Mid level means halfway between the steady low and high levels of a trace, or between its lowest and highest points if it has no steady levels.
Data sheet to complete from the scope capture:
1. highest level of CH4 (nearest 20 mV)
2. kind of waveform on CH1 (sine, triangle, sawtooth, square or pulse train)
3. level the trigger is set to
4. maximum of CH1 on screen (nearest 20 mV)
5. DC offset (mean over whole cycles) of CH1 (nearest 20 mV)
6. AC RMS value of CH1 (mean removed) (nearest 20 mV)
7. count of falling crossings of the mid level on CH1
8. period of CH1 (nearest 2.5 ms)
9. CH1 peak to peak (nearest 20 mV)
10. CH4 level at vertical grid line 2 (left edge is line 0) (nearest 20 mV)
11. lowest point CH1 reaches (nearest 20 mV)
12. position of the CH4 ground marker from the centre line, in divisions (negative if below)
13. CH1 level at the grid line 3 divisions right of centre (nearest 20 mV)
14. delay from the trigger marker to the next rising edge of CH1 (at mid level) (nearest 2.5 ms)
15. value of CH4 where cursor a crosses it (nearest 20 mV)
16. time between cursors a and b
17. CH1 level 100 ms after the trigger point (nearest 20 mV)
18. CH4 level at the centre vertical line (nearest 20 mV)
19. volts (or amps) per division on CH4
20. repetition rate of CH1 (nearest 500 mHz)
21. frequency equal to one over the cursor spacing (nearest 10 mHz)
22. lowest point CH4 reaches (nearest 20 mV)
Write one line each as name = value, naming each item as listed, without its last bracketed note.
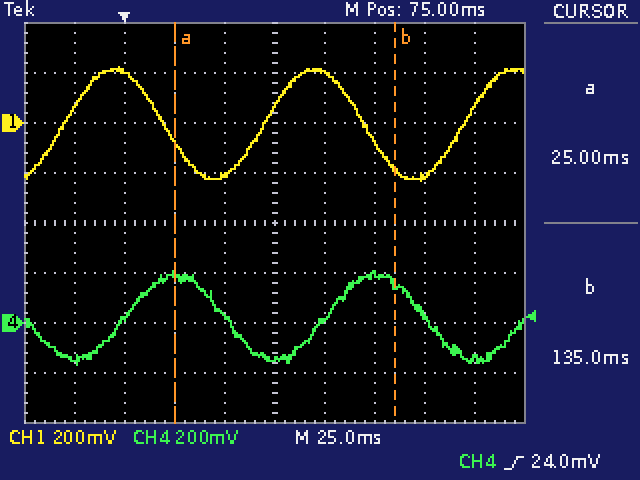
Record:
highest level of CH4 = 200 mV
kind of waveform on CH1 = sine
level the trigger is set to = 24.0 mV
maximum of CH1 on screen = 220 mV
DC offset (mean over whole cycles) of CH1 = 0 mV
AC RMS value of CH1 (mean removed) = 160 mV
count of falling crossings of the mid level on CH1 = 2
period of CH1 = 100.0 ms
CH1 peak to peak = 460 mV
CH4 level at vertical grid line 2 (left edge is line 0) = 20 mV
lowest point CH1 reaches = -240 mV
position of the CH4 ground marker from the centre line, in divisions = -2.0 div
CH1 level at the grid line 3 divisions right of centre = -220 mV
delay from the trigger marker to the next rising edge of CH1 (at mid level) = 70.0 ms
value of CH4 where cursor a crosses it = 180 mV
time between cursors a and b = 110.0 ms
CH1 level 100 ms after the trigger point = 200 mV
CH4 level at the centre vertical line = -140 mV
volts (or amps) per division on CH4 = 200 mV
repetition rate of CH1 = 10.0 Hz
frequency equal to one over the cursor spacing = 9.09 Hz
lowest point CH4 reaches = -160 mV
